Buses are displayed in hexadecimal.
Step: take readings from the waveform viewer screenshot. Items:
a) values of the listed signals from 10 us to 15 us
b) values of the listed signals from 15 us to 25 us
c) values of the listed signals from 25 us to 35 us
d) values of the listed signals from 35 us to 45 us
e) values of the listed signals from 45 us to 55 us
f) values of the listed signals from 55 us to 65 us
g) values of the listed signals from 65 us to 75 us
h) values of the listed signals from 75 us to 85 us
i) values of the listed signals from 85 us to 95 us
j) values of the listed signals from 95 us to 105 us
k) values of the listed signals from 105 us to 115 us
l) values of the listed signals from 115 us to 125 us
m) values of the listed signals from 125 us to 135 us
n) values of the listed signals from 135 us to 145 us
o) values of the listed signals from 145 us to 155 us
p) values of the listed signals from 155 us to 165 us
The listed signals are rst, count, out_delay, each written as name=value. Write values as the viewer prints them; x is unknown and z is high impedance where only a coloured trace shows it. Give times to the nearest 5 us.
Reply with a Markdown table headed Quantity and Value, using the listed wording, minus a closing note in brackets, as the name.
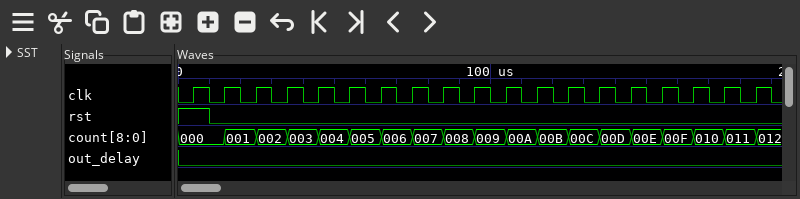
| Quantity | Value |
|---|---|
| values of the listed signals from 10 us to 15 us | rst=0, count=000, out_delay=0 |
| values of the listed signals from 15 us to 25 us | rst=0, count=001, out_delay=0 |
| values of the listed signals from 25 us to 35 us | rst=0, count=002, out_delay=0 |
| values of the listed signals from 35 us to 45 us | rst=0, count=003, out_delay=0 |
| values of the listed signals from 45 us to 55 us | rst=0, count=004, out_delay=0 |
| values of the listed signals from 55 us to 65 us | rst=0, count=005, out_delay=0 |
| values of the listed signals from 65 us to 75 us | rst=0, count=006, out_delay=0 |
| values of the listed signals from 75 us to 85 us | rst=0, count=007, out_delay=0 |
| values of the listed signals from 85 us to 95 us | rst=0, count=008, out_delay=0 |
| values of the listed signals from 95 us to 105 us | rst=0, count=009, out_delay=0 |
| values of the listed signals from 105 us to 115 us | rst=0, count=00A, out_delay=0 |
| values of the listed signals from 115 us to 125 us | rst=0, count=00B, out_delay=0 |
| values of the listed signals from 125 us to 135 us | rst=0, count=00C, out_delay=0 |
| values of the listed signals from 135 us to 145 us | rst=0, count=00D, out_delay=0 |
| values of the listed signals from 145 us to 155 us | rst=0, count=00E, out_delay=0 |
| values of the listed signals from 155 us to 165 us | rst=0, count=00F, out_delay=0 |
